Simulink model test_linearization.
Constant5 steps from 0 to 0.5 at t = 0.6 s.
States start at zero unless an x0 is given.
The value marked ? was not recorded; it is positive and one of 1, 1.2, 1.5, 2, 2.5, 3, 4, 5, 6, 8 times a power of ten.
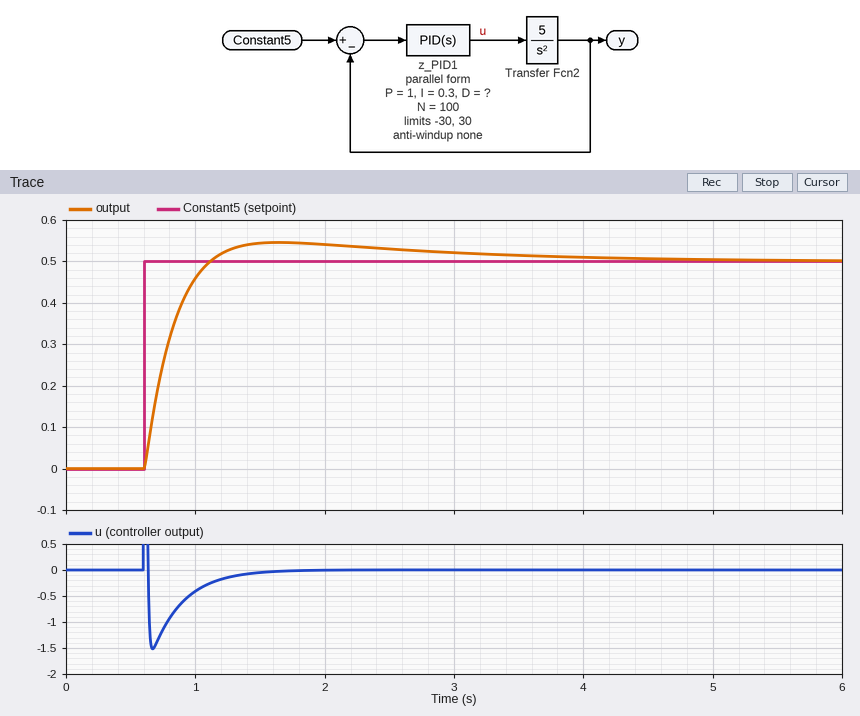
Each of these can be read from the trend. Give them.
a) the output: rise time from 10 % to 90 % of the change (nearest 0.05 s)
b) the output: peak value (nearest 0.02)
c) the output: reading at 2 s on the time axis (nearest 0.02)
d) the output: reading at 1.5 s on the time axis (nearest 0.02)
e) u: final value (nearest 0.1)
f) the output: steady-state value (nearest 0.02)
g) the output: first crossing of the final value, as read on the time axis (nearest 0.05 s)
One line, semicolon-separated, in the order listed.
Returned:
0.35 s; 0.54; 0.54; 0.54; 0.0; 0.50; 1.10 s
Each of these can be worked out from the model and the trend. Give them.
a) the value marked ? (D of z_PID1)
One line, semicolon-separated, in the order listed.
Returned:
1
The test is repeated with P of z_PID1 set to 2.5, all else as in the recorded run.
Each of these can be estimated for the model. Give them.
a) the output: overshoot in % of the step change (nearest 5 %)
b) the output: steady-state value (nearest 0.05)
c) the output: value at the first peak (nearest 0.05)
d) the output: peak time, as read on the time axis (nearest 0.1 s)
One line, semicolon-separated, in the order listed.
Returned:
20 %; 0.50; 0.60; 1.3 s
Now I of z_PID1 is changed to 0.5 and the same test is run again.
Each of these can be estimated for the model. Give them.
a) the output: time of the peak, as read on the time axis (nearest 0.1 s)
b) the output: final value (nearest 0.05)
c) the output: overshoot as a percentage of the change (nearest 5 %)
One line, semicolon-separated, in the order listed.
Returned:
1.7 s; 0.50; 10 %
